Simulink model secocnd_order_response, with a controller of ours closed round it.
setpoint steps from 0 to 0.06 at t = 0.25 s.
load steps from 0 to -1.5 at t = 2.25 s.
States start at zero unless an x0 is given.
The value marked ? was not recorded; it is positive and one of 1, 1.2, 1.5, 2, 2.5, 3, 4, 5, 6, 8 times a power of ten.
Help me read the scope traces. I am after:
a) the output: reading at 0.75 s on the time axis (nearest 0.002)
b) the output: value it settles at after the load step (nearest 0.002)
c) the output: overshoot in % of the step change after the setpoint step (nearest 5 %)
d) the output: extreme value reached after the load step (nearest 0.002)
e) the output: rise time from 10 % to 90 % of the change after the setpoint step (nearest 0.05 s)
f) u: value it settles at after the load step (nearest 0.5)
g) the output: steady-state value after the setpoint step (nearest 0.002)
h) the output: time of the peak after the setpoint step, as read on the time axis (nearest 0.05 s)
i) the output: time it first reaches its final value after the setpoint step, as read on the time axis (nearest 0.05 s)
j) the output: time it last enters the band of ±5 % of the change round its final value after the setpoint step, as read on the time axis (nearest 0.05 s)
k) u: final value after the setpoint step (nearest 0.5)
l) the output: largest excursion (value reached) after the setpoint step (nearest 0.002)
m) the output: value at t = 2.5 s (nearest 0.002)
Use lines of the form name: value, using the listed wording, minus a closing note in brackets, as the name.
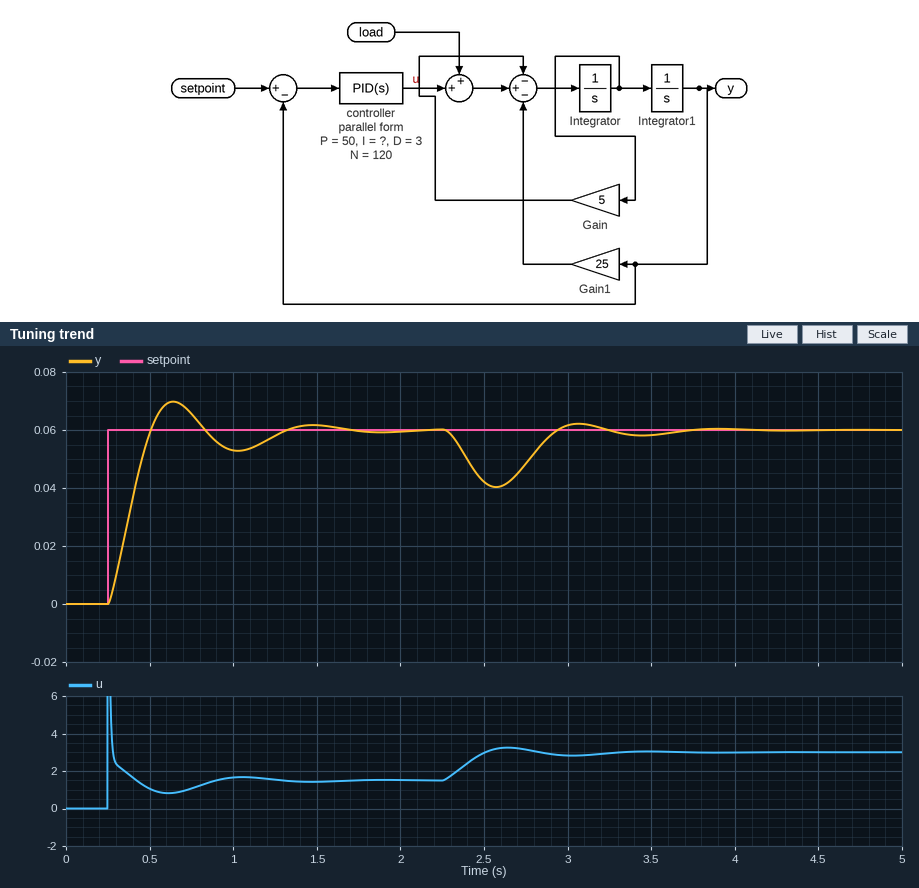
the output: reading at 0.75 s on the time axis: 0.066
the output: value it settles at after the load step: 0.060
the output: overshoot in % of the step change after the setpoint step: 15 %
the output: extreme value reached after the load step: 0.040
the output: rise time from 10 % to 90 % of the change after the setpoint step: 0.20 s
u: value it settles at after the load step: 3.0
the output: steady-state value after the setpoint step: 0.060
the output: time of the peak after the setpoint step, as read on the time axis: 0.65 s
the output: time it first reaches its final value after the setpoint step, as read on the time axis: 0.50 s
the output: time it last enters the band of ±5 % of the change round its final value after the setpoint step, as read on the time axis: 1.20 s
u: final value after the setpoint step: 1.5
the output: largest excursion (value reached) after the setpoint step: 0.070
the output: value at t = 2.5 s: 0.042
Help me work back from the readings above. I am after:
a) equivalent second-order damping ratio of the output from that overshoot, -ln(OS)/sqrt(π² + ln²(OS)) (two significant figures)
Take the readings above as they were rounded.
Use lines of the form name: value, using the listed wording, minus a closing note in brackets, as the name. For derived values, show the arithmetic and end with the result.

equivalent second-order damping ratio of the output from that overshoot, -ln(OS)/sqrt(π² + ln²(OS)): ln(0.15) = -1.897; 1.897 / sqrt(9.870 + 3.599) = 0.52
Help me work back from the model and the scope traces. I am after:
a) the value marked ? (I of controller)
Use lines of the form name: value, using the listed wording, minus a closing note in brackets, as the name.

the value marked ?: 200
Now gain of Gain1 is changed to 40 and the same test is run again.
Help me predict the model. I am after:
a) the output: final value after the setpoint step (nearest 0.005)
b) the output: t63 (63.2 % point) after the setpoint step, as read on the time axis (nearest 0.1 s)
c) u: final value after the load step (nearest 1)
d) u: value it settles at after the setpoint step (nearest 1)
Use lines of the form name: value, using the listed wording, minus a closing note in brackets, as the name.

the output: final value after the setpoint step: 0.060
the output: t63 (63.2 % point) after the setpoint step, as read on the time axis: 0.4 s
u: final value after the load step: 4
u: value it settles at after the setpoint step: 2
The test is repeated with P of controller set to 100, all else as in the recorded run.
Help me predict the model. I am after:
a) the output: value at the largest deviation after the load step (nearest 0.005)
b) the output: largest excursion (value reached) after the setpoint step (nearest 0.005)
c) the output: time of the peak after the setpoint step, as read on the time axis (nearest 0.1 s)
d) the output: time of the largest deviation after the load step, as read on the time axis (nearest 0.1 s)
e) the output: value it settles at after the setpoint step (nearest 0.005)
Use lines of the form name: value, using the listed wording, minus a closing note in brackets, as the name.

the output: value at the largest deviation after the load step: 0.045
the output: largest excursion (value reached) after the setpoint step: 0.075
the output: time of the peak after the setpoint step, as read on the time axis: 0.5 s
the output: time of the largest deviation after the load step, as read on the time axis: 2.5 s
the output: value it settles at after the setpoint step: 0.060
